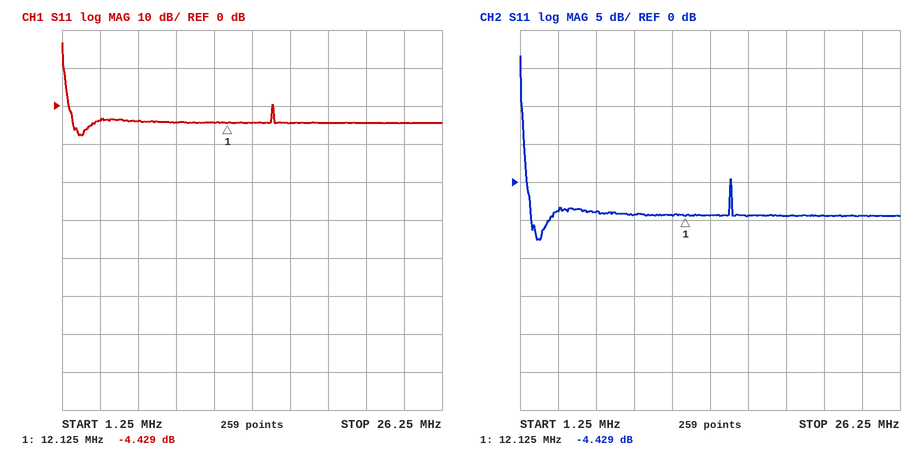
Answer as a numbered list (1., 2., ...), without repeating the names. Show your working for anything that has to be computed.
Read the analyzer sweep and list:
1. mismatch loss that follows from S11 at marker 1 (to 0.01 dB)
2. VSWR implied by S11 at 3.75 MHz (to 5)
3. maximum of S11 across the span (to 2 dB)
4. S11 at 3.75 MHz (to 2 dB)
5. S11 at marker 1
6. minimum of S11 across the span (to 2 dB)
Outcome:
1. −10 log10(1 − 10^(-4.429/10)) ≈ 1.94 dB
2. |Γ| = 10^(-4/20) = 0.6310; VSWR = (1 + 0.6310)/(1 − 0.6310) ≈ 4.42, so 5 to the nearest 5
3. 16 dB
4. -4 dB
5. -4.429 dB
6. -8 dB
